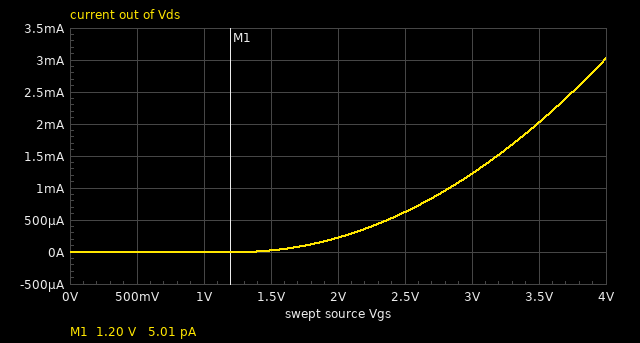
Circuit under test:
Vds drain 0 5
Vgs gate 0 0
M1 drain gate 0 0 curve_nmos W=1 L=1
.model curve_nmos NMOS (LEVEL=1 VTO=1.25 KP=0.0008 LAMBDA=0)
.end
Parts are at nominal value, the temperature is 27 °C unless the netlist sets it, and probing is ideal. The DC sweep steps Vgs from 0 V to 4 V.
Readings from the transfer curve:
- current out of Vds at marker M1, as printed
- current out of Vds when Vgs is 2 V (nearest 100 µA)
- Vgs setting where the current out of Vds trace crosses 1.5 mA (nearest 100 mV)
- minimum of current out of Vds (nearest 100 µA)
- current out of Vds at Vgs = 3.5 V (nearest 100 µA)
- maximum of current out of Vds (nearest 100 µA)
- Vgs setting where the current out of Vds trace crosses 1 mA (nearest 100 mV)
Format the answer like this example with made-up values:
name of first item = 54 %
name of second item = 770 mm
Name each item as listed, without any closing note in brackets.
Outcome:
current out of Vds at marker M1, as printed = 5.01 pA
current out of Vds when Vgs is 2 V = 200 µA
Vgs setting where the current out of Vds trace crosses 1.5 mA = 3.2 V
minimum of current out of Vds = 0 A
current out of Vds at Vgs = 3.5 V = 2.0 mA
maximum of current out of Vds = 3.0 mA
Vgs setting where the current out of Vds trace crosses 1 mA = 2.8 V
